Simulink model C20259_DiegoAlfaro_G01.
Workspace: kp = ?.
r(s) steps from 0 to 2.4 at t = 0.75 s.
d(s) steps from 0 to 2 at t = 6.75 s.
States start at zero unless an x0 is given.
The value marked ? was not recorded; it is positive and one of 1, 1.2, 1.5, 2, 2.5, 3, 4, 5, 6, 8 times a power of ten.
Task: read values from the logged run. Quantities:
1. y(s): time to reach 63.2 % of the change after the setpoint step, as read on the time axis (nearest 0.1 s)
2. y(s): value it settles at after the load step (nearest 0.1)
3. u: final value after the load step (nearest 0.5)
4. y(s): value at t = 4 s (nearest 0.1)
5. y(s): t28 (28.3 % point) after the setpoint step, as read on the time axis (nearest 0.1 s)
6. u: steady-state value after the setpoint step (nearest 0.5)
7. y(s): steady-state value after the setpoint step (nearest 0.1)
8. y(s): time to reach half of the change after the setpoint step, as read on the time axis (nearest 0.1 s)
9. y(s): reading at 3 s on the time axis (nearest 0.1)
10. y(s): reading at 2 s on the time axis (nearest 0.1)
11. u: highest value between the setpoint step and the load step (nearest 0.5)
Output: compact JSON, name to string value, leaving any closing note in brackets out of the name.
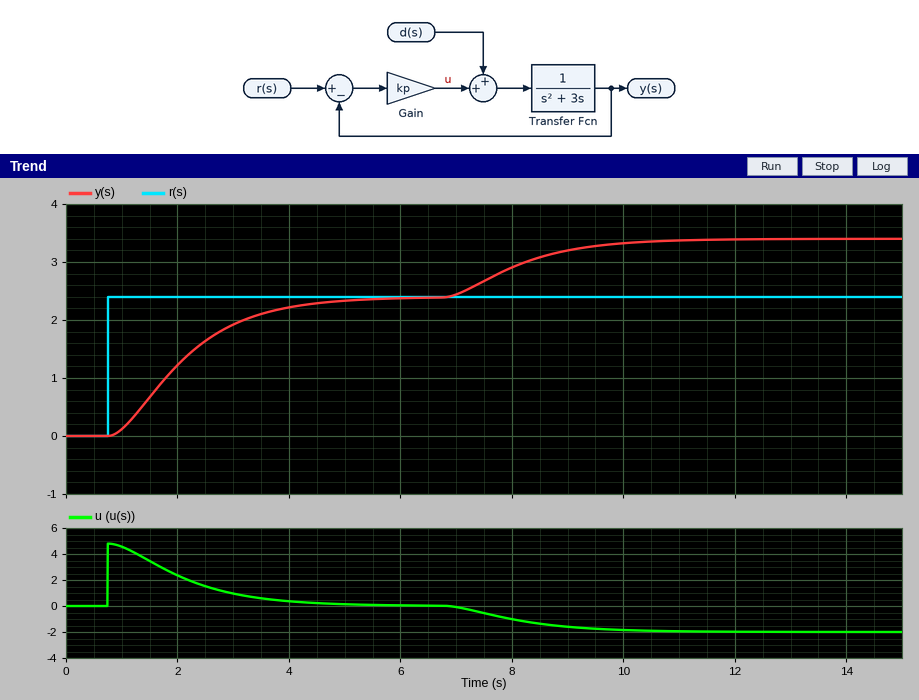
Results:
{"y(s): time to reach 63.2 % of the change after the setpoint step, as read on the time axis": "2.3 s", "y(s): value it settles at after the load step": "3.4", "u: final value after the load step": "-2.0", "y(s): value at t = 4 s": "2.2", "y(s): t28 (28.3 % point) after the setpoint step, as read on the time axis": "1.5 s", "u: steady-state value after the setpoint step": "0.0", "y(s): steady-state value after the setpoint step": "2.4", "y(s): time to reach half of the change after the setpoint step, as read on the time axis": "2.0 s", "y(s): reading at 3 s on the time axis": "1.9", "y(s): reading at 2 s on the time axis": "1.2", "u: highest value between the setpoint step and the load step": "5.0"}
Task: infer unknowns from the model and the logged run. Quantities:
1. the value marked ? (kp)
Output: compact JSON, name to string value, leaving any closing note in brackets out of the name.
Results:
{"the value marked ?": "2"}
